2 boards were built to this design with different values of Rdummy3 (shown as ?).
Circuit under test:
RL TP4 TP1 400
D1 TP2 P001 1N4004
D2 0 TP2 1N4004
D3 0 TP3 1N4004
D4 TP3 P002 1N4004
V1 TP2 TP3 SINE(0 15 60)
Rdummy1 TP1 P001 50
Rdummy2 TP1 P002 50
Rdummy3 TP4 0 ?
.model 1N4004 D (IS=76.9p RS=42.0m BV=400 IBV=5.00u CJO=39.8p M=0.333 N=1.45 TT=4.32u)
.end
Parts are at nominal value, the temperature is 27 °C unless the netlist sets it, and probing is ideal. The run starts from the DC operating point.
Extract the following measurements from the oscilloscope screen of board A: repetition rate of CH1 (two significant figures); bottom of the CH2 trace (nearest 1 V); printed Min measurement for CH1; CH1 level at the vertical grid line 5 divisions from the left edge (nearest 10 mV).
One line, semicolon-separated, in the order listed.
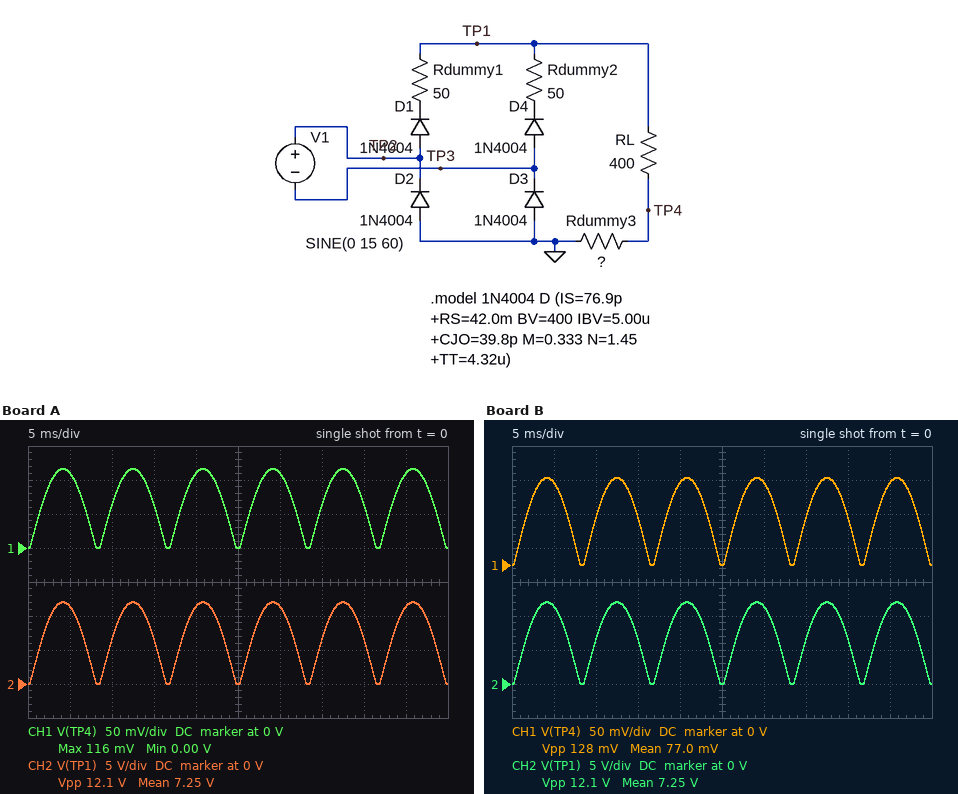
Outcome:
120 Hz; 0 V; 0.00 V; 0 V
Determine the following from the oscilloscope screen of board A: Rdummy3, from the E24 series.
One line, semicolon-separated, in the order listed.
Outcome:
3.9 Ω
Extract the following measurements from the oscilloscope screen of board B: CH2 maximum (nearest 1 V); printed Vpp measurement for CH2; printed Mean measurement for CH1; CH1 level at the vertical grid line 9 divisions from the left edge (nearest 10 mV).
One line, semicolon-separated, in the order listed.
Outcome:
12 V; 12.1 V; 77.0 mV; 120 mV
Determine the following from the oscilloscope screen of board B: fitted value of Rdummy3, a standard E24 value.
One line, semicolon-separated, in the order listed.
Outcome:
4.3 Ω
